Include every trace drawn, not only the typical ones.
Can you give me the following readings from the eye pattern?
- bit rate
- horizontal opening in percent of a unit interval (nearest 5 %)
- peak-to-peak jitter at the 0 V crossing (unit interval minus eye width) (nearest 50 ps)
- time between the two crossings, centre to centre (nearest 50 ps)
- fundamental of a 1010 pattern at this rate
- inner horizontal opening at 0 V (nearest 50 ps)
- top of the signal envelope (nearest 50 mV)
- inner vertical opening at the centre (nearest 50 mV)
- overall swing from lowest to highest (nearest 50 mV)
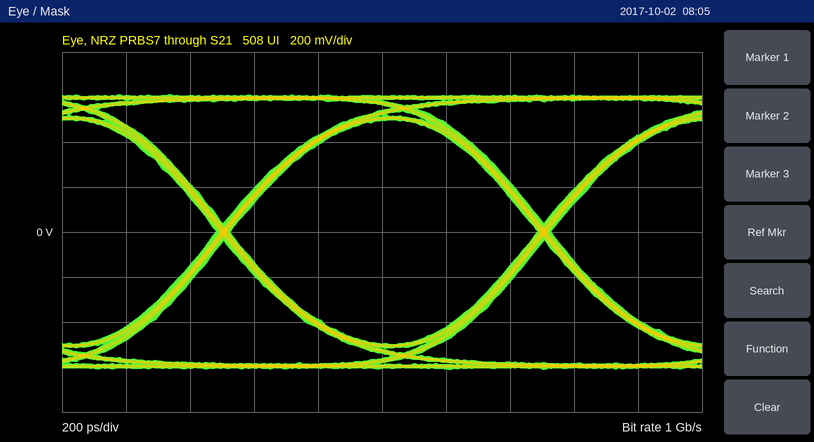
1 Gb/s
95 %
50 ps
1.00 ns
500 MHz
950 ps
600 mV
1.00 V
1.20 V
